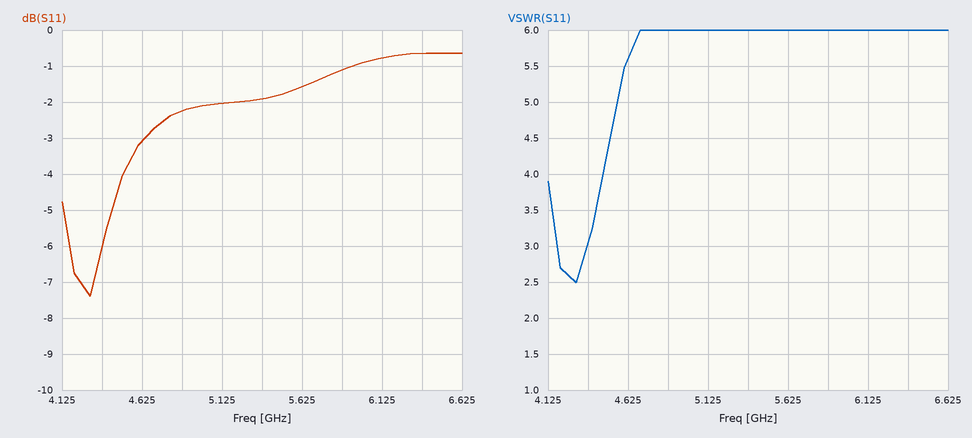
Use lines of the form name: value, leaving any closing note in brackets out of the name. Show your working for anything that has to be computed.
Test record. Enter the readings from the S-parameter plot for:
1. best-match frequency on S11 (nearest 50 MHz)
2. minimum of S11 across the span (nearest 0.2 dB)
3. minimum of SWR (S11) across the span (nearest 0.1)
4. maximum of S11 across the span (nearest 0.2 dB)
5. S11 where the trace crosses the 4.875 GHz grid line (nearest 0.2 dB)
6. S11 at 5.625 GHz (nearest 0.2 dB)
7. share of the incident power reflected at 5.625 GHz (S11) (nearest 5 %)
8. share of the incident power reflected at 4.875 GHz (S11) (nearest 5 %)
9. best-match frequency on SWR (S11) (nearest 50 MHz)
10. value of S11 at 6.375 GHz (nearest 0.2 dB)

best-match frequency on S11: 4.30 GHz
minimum of S11 across the span: -7.4 dB
minimum of SWR (S11) across the span: 2.5
maximum of S11 across the span: -0.6 dB
S11 where the trace crosses the 4.875 GHz grid line: -2.2 dB
S11 at 5.625 GHz: -1.6 dB
share of the incident power reflected at 5.625 GHz (S11): 10^(-1.6/10) ≈ 69.2 %, so 70 % to the nearest 5 %
share of the incident power reflected at 4.875 GHz (S11): 10^(-2.2/10) ≈ 60 %
best-match frequency on SWR (S11): 4.30 GHz
value of S11 at 6.375 GHz: -0.6 dB
